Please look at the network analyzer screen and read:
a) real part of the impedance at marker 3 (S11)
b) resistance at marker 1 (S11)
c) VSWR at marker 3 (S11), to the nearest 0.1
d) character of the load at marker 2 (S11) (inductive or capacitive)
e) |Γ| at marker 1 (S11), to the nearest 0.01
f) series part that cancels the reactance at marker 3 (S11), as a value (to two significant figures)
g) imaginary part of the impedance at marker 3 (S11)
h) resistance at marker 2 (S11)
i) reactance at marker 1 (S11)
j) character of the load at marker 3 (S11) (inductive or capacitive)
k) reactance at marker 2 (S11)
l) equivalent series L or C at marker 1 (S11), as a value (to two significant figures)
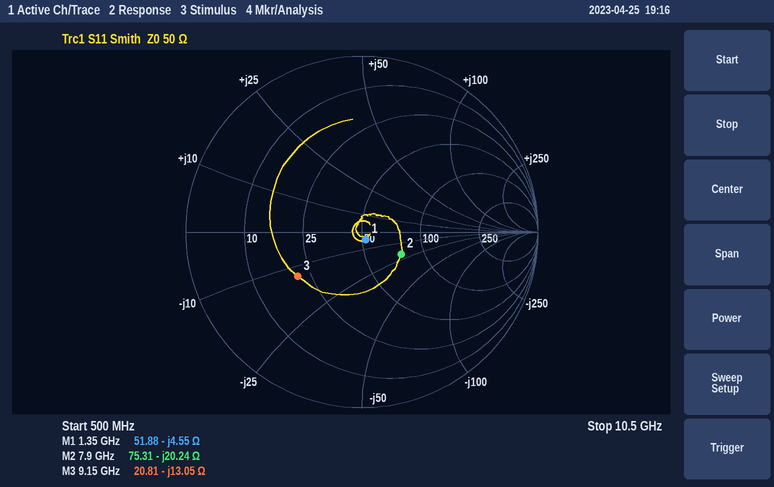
20.81 Ω
51.88 Ω
2.6
capacitive
0.05
230 pH
-13.05 Ω
75.31 Ω
-4.55 Ω
capacitive
-20.24 Ω
26 pF
